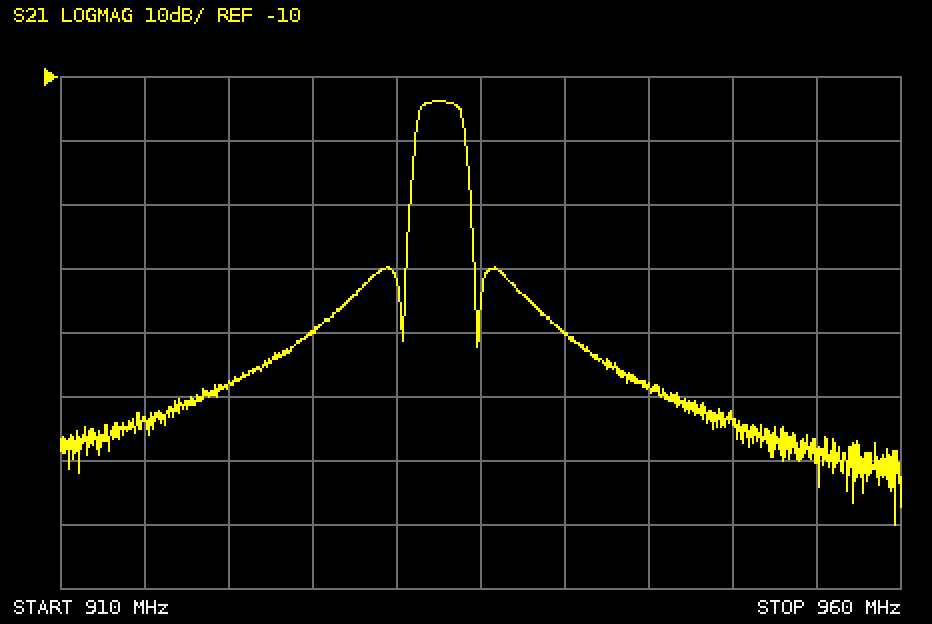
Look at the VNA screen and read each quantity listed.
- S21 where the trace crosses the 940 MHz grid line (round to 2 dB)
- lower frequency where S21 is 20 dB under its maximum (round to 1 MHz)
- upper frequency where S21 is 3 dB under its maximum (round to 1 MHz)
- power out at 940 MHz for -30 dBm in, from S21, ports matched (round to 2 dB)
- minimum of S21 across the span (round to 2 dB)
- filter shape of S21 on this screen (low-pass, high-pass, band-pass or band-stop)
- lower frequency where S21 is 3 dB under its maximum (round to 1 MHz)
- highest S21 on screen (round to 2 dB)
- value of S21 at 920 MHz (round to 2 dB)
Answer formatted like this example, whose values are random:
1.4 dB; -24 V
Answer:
-50 dB; 931 MHz; 934 MHz; -80 dBm; -80 dB; band-pass; 931 MHz; -14 dB; -58 dB
